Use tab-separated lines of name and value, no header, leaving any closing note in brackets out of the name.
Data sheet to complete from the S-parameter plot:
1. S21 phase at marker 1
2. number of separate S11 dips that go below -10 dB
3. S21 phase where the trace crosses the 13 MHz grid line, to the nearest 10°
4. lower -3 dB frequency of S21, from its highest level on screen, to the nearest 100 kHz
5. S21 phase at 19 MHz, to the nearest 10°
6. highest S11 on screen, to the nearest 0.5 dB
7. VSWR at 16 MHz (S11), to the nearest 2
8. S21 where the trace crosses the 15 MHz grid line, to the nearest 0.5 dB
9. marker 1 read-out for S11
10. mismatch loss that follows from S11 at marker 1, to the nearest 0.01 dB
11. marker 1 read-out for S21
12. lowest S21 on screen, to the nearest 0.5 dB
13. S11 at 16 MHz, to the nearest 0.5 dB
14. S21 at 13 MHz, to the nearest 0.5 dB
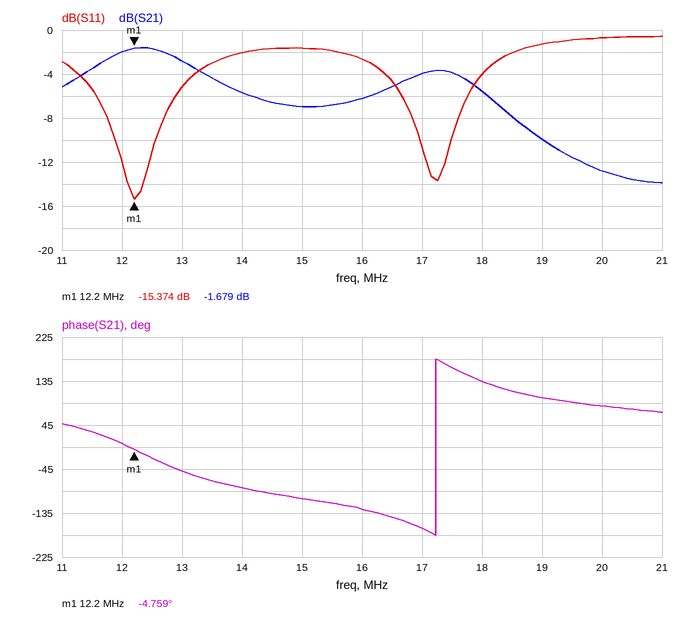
S21 phase at marker 1	-4.759°
number of separate S11 dips that go below -10 dB	2
S21 phase where the trace crosses the 13 MHz grid line, to the nearest 10°	-50°
lower -3 dB frequency of S21, from its highest level on screen, to the nearest 100 kHz	11.2 MHz
S21 phase at 19 MHz, to the nearest 10°	100°
highest S11 on screen, to the nearest 0.5 dB	-0.5 dB
VSWR at 16 MHz (S11), to the nearest 2	6
S21 where the trace crosses the 15 MHz grid line, to the nearest 0.5 dB	-7.0 dB
marker 1 read-out for S11	-15.374 dB
mismatch loss that follows from S11 at marker 1, to the nearest 0.01 dB	0.13 dB
marker 1 read-out for S21	-1.679 dB
lowest S21 on screen, to the nearest 0.5 dB	-14.0 dB
S11 at 16 MHz, to the nearest 0.5 dB	-2.5 dB
S21 at 13 MHz, to the nearest 0.5 dB	-3.0 dB
